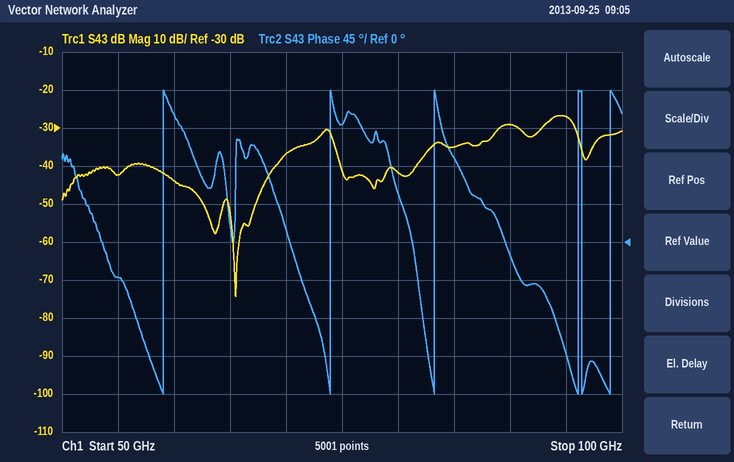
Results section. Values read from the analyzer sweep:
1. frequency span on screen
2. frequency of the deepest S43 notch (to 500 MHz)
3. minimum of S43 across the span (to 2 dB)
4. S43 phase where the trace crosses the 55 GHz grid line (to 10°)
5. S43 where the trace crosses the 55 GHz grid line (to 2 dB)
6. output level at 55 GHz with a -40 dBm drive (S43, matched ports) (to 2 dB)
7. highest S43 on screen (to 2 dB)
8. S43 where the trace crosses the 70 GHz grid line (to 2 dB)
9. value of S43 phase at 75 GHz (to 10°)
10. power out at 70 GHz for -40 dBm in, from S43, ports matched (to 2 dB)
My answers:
50 GHz
65.5 GHz
-74 dB
-40°
-42 dB
-82 dBm
-26 dB
-36 dB
140°
-76 dBm
